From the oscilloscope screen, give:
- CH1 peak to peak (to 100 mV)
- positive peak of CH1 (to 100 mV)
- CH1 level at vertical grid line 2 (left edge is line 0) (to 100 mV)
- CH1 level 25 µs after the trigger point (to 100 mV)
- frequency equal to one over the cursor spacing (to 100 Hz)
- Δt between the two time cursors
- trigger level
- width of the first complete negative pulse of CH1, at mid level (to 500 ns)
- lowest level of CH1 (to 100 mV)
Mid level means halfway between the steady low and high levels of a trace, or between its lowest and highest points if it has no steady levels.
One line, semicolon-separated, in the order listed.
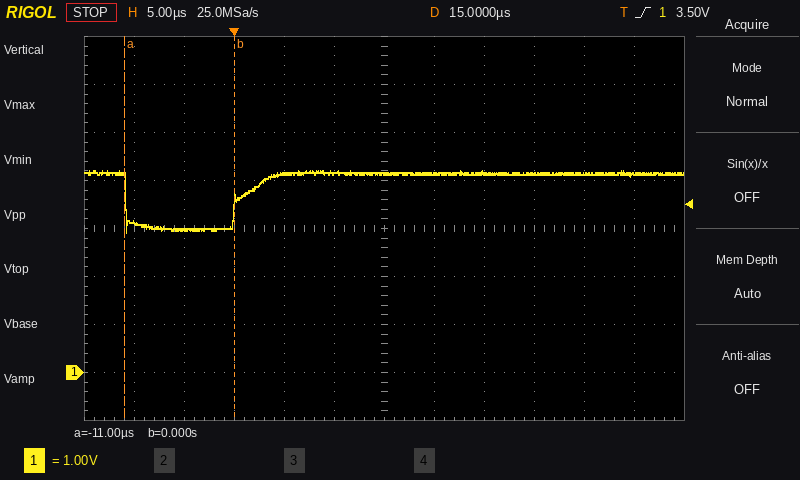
1.3 V; 4.2 V; 3.0 V; 4.2 V; 90.9 kHz; 11.0 µs; 3.50 V; 11.0 µs; 2.9 V
